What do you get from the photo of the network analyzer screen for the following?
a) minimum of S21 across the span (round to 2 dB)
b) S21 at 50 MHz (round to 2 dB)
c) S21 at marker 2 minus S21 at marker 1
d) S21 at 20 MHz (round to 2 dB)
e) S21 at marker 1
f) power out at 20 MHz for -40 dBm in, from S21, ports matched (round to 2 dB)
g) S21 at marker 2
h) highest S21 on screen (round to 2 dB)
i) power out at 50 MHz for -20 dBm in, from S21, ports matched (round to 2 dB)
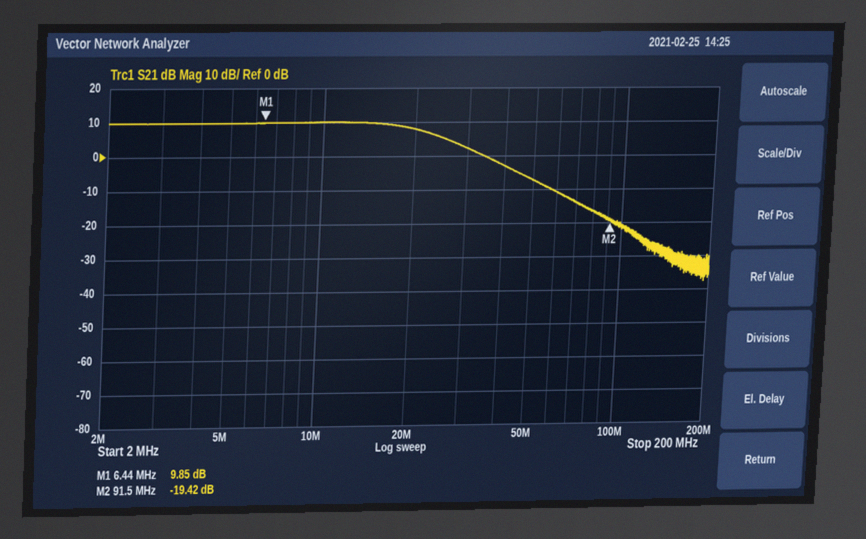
-38 dB
-8 dB
-29.27 dB
8 dB
9.85 dB
-32 dBm
-19.42 dB
10 dB
-28 dBm
